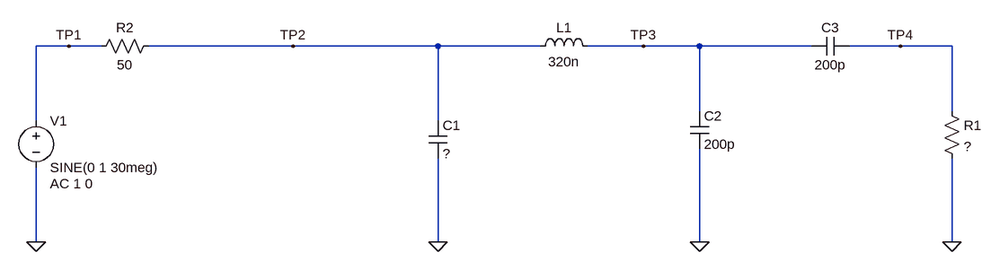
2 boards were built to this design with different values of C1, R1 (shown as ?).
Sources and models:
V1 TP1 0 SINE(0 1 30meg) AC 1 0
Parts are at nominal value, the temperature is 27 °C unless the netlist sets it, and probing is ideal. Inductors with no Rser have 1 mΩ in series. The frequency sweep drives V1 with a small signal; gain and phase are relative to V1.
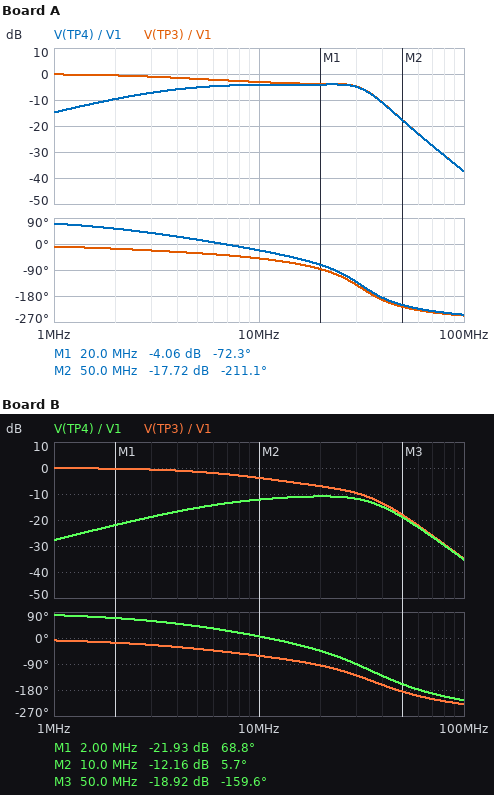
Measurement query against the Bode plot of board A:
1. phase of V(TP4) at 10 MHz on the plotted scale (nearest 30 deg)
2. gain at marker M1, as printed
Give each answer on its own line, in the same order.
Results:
-30 deg
-4.06 dB
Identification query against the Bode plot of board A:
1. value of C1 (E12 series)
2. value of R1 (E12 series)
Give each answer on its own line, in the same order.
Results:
100 pF
150 Ω
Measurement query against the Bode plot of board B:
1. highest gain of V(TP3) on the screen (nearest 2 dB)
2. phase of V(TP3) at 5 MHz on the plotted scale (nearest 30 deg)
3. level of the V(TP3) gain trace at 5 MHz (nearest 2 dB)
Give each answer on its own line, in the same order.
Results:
0 dB
-30 deg
-2 dB
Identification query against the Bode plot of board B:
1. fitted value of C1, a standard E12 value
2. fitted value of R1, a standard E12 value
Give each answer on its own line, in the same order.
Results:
68 pF
33 Ω
